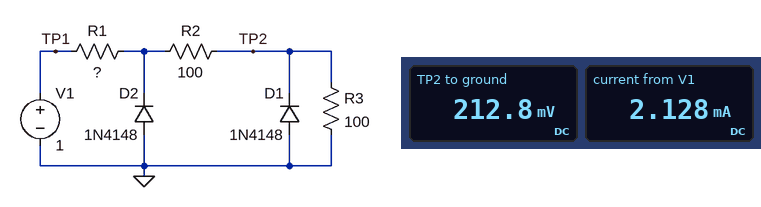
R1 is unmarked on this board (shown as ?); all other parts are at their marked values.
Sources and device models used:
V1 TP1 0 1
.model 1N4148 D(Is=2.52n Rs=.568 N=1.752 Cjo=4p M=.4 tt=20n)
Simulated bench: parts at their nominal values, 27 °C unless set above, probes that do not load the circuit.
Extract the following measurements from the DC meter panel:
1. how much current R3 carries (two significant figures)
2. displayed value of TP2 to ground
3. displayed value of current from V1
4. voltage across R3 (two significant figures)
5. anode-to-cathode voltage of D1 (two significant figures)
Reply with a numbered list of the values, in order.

1. 2.1 mA
2. 212.8 mV
3. 2.128 mA
4. 210 mV
5. -210 mV
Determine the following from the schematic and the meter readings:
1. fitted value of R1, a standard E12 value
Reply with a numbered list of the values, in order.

1. 270 Ω
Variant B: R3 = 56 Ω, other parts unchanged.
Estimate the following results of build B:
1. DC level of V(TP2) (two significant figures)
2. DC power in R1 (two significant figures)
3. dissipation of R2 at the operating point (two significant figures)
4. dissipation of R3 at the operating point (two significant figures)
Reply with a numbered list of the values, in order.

1. 130 mV
2. 1.5 mW
3. 550 µW
4. 310 µW
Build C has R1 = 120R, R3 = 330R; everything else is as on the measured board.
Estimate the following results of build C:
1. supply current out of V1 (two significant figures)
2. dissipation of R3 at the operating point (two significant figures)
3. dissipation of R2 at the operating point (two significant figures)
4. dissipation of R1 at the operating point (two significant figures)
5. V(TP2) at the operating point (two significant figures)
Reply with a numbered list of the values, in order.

1. 1.8 mA
2. 1.1 mW
3. 330 µW
4. 400 µW
5. 600 mV
